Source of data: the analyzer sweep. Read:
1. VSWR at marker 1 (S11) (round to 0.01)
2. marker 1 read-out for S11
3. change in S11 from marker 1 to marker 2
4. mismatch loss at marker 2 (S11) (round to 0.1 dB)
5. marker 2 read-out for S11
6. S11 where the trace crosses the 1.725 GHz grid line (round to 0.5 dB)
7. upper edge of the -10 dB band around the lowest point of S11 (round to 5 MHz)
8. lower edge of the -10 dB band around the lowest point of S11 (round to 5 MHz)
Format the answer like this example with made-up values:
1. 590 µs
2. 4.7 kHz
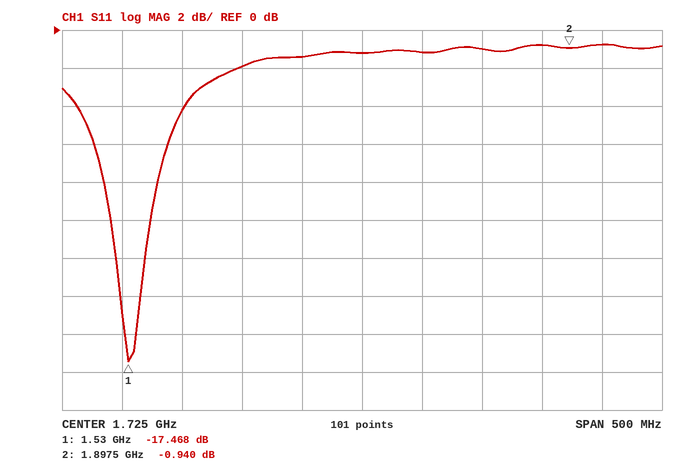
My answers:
1. 1.31
2. -17.468 dB
3. 16.528 dB
4. 7.1 dB
5. -0.940 dB
6. -1.0 dB
7. 1.550 GHz
8. 1.515 GHz
